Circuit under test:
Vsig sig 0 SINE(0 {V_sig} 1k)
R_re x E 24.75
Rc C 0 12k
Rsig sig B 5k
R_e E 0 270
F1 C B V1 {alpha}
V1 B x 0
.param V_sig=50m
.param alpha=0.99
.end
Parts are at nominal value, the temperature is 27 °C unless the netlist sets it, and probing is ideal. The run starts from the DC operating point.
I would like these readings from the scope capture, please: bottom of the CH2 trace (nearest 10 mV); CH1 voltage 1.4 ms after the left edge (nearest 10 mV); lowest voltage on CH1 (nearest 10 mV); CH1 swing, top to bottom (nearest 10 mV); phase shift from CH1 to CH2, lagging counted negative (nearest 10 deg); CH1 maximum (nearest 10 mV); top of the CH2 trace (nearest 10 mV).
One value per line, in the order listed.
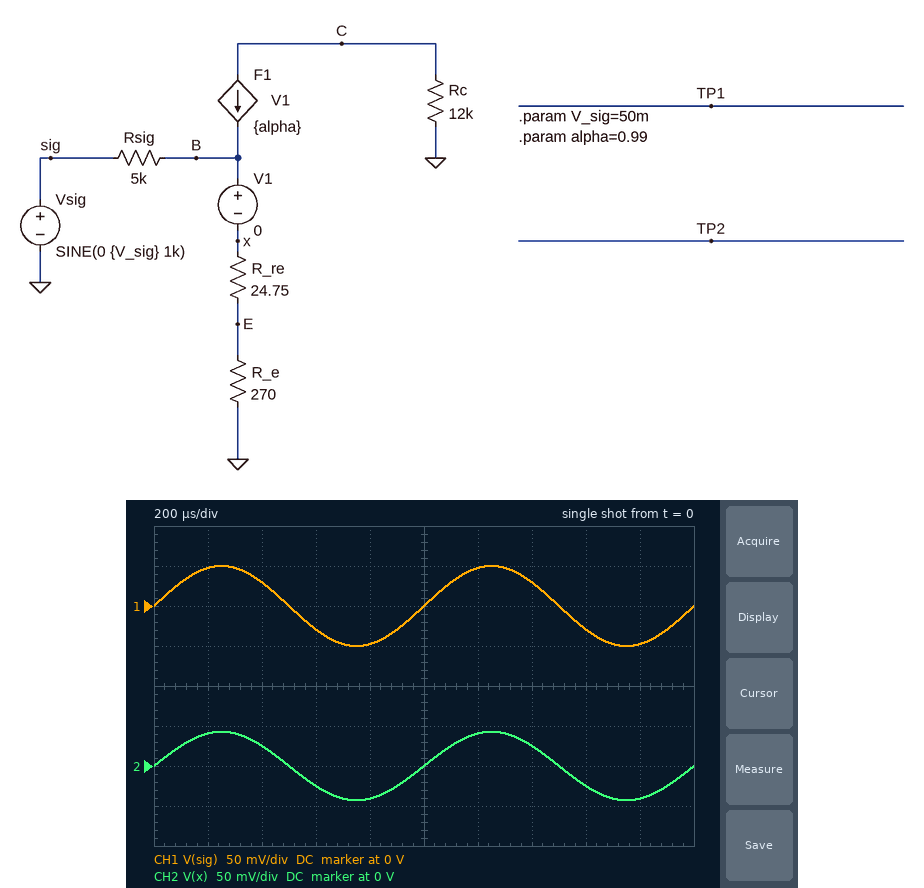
-40 mV
30 mV
-50 mV
100 mV
0 deg
50 mV
40 mV
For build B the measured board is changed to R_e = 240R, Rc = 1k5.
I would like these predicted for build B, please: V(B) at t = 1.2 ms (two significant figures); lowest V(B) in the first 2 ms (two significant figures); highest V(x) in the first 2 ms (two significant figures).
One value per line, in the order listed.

40 mV
-42 mV
42 mV
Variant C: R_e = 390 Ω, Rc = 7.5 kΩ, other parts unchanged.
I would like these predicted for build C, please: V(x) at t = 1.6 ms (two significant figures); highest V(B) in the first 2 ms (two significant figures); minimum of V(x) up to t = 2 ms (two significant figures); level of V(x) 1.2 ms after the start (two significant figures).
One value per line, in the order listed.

-26 mV
45 mV
-45 mV
42 mV
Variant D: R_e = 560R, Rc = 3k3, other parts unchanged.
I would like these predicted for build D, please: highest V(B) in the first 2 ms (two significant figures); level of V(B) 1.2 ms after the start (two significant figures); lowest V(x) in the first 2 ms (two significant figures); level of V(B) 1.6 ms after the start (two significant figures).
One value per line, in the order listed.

46 mV
44 mV
-46 mV
-27 mV
